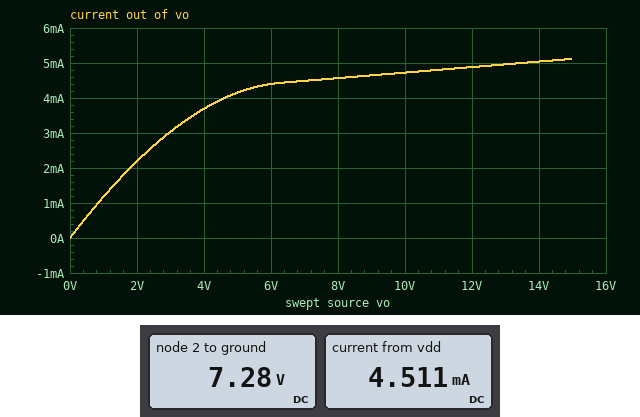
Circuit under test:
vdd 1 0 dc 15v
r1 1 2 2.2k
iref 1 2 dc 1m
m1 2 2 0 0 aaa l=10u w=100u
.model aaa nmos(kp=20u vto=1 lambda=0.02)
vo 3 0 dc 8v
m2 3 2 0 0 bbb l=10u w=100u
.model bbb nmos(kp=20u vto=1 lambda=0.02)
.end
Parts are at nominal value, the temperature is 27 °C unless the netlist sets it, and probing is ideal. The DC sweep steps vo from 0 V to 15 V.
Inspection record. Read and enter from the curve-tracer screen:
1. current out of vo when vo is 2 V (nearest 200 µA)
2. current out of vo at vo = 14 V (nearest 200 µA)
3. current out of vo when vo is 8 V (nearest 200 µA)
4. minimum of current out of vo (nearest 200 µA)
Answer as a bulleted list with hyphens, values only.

- 2.2 mA
- 5.0 mA
- 4.6 mA
- 0 A
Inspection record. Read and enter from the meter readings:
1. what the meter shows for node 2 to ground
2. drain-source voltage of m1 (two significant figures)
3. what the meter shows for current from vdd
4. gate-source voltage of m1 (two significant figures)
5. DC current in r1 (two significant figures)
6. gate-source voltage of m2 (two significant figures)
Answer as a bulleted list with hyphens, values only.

- 7.28 V
- 7.3 V
- 4.511 mA
- 7.3 V
- 3.5 mA
- 7.3 V
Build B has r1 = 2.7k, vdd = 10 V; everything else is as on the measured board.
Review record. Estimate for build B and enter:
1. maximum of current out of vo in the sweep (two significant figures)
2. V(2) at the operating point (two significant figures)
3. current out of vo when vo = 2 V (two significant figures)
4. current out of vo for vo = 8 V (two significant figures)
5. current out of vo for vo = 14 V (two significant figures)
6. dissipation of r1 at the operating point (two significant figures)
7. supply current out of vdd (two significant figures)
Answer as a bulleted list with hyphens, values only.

- 3.0 mA
- 5.8 V
- 1.6 mA
- 2.7 mA
- 2.9 mA
- 6.6 mW
- 2.6 mA
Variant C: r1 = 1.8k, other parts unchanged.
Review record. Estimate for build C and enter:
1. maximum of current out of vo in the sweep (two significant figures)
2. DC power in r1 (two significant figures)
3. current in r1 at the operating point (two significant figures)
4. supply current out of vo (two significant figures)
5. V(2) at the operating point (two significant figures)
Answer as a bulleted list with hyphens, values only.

- 5.7 mA
- 30 mW
- 4.1 mA
- 5.1 mA
- 7.6 V
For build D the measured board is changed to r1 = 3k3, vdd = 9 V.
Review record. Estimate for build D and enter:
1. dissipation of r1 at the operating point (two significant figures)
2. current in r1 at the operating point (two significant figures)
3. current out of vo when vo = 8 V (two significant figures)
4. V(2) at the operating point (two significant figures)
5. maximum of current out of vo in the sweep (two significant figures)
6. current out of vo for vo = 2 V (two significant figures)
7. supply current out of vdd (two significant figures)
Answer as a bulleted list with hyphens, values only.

- 4.0 mW
- 1.1 mA
- 2.2 mA
- 5.4 V
- 2.5 mA
- 1.4 mA
- 2.1 mA
